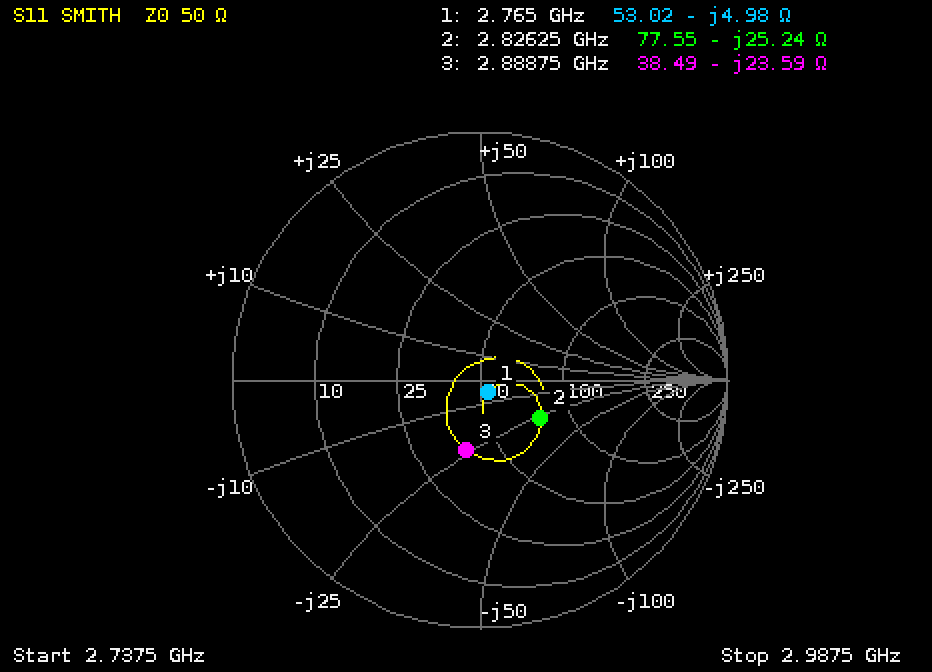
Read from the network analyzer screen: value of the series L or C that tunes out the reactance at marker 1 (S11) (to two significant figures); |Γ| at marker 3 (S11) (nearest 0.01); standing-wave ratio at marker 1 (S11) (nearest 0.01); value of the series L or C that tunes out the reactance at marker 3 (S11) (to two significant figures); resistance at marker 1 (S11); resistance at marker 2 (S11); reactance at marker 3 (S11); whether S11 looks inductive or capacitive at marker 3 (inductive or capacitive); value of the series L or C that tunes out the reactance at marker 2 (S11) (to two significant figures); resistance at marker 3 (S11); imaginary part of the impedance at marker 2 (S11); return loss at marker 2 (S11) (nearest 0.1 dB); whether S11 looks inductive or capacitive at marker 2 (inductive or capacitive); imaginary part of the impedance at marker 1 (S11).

290 pH
0.29
1.12
1.3 nH
53.02 Ω
77.55 Ω
-23.59 Ω
capacitive
1.4 nH
38.49 Ω
-25.24 Ω
10.8 dB
capacitive
-4.98 Ω
